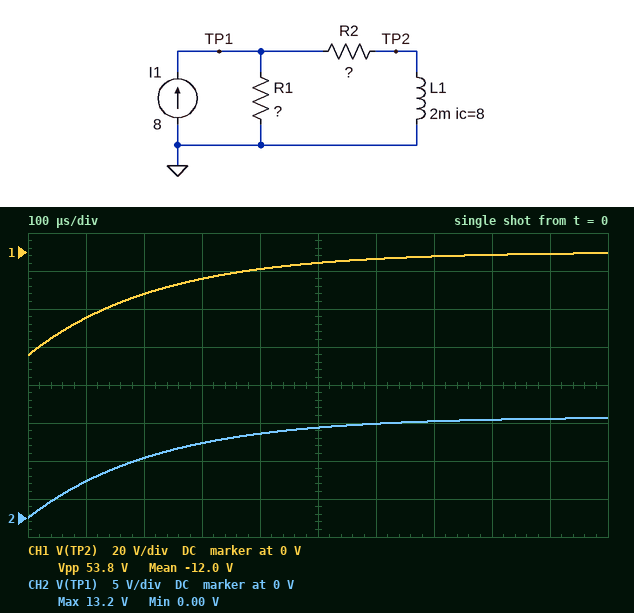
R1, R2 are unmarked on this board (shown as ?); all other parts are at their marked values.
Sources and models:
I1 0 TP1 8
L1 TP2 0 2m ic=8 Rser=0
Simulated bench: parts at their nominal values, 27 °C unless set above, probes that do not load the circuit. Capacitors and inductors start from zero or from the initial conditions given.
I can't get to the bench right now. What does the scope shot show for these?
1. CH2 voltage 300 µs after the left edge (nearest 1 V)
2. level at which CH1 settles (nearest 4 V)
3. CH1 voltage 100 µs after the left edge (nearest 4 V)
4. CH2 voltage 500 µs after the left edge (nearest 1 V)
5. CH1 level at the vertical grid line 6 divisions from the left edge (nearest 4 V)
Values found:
10 V
0 V
-36 V
12 V
-4 V
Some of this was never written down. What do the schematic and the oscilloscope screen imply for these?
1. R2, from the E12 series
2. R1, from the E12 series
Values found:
6.8 Ω
2.2 Ω
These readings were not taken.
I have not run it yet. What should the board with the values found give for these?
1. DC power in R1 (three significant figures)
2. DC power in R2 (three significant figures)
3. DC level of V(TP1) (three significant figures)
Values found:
80.4 W
26.0 W
13.3 V
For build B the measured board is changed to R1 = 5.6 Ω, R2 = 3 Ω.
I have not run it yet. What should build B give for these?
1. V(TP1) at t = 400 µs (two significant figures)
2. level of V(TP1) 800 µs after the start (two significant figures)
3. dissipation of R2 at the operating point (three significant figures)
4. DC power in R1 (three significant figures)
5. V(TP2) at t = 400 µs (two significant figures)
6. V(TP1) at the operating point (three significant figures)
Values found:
13 V
15 V
81.4 W
43.6 W
-4.3 V
15.6 V
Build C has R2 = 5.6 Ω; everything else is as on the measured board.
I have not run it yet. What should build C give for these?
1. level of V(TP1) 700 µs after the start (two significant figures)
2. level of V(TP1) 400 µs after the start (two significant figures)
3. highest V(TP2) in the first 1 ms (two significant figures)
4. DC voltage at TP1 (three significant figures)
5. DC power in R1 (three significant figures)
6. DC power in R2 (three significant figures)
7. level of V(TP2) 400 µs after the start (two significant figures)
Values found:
12 V
10 V
-910 mV
12.6 V
72.6 W
28.5 W
-9.4 V
